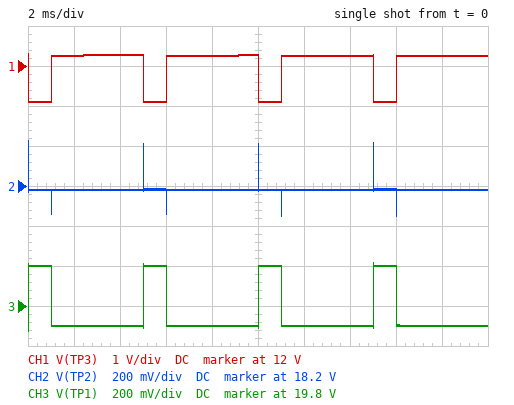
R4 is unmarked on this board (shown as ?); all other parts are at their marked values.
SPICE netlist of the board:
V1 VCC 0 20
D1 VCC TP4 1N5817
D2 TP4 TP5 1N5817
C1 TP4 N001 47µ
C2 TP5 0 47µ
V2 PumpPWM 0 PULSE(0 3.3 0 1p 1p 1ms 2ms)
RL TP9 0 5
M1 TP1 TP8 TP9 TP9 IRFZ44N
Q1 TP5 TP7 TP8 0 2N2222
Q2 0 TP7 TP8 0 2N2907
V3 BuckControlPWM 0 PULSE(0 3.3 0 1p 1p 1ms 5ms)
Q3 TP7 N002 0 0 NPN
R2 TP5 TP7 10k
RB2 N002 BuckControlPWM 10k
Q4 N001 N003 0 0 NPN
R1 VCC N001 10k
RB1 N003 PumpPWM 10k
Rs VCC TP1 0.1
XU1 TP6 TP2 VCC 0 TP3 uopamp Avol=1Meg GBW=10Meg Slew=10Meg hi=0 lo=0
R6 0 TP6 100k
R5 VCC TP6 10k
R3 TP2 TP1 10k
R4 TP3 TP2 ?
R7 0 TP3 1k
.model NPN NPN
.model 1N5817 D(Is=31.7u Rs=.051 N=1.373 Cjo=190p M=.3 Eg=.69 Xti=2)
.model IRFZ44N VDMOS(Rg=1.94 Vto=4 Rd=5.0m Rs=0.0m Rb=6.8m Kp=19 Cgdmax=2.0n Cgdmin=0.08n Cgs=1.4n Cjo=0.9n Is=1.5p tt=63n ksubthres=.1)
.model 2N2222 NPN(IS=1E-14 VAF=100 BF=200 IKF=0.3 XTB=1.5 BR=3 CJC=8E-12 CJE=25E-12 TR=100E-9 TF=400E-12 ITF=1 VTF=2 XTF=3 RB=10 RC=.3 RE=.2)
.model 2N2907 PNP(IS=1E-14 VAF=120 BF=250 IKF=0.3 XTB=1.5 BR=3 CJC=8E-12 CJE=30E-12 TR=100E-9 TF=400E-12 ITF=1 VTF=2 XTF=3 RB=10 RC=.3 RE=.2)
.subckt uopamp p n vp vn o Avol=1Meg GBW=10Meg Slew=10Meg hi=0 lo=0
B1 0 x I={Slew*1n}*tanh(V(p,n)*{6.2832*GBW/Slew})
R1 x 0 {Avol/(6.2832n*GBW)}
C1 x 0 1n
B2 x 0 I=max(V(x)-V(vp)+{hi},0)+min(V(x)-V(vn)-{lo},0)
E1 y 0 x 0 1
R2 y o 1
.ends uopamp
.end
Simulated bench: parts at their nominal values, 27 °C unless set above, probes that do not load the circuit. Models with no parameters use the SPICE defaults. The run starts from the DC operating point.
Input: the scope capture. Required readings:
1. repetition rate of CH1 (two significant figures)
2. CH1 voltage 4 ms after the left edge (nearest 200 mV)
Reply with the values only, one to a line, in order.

200 Hz
12.2 V
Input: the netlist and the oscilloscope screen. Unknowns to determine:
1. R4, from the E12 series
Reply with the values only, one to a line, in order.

39 kΩ
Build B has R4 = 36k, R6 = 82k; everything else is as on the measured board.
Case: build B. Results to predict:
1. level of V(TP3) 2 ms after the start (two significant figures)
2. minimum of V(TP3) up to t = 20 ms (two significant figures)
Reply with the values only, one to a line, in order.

11 V
10 V
